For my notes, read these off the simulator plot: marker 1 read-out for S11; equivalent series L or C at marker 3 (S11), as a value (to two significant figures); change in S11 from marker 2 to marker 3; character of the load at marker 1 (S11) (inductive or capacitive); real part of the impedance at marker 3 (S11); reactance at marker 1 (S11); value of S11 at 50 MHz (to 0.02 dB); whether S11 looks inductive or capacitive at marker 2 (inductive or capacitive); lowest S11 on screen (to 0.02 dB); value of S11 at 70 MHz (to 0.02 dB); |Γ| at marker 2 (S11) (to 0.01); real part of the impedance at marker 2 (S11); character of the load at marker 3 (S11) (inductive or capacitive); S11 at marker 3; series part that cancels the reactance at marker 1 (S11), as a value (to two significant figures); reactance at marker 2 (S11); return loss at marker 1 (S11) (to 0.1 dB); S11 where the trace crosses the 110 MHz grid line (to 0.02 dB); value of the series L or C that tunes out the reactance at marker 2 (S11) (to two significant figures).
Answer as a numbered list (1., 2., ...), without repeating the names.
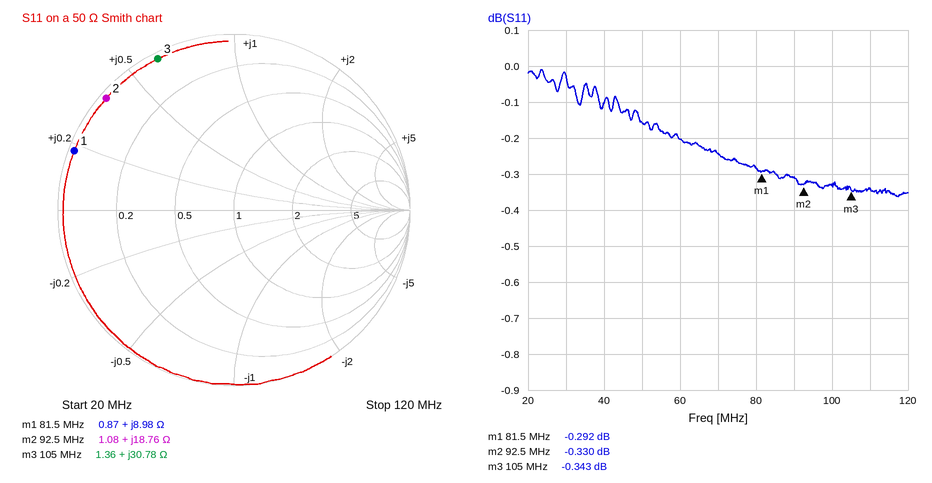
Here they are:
1. -0.292 dB
2. 47 nH
3. -0.013 dB
4. inductive
5. 1.36 Ω
6. +8.98 Ω
7. -0.16 dB
8. inductive
9. -0.36 dB
10. -0.24 dB
11. 0.96
12. 1.08 Ω
13. inductive
14. -0.343 dB
15. 220 pF
16. +18.76 Ω
17. 0.3 dB
18. -0.34 dB
19. 92 pF
